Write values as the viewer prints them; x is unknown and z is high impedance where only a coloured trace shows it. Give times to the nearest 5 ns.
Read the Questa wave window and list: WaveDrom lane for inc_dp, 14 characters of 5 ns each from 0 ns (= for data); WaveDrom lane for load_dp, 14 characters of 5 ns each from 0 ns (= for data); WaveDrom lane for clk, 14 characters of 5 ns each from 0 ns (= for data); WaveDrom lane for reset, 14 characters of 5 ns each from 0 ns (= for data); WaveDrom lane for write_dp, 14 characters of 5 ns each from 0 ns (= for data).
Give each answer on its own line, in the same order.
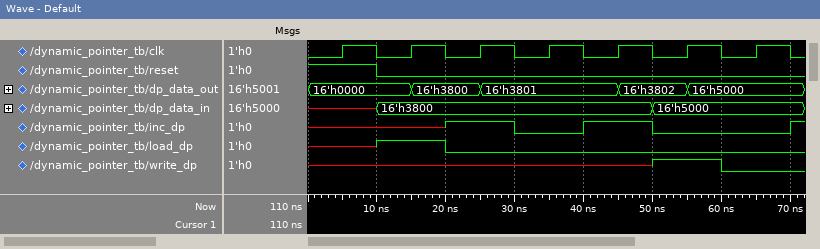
{name: 'inc_dp', wave: 'x...1.0.1.0...'}
{name: 'load_dp', wave: 'x.1.0.........'}
{name: 'clk', wave: '01010101010101'}
{name: 'reset', wave: '1.0...........'}
{name: 'write_dp', wave: 'x.........1.0.'}
